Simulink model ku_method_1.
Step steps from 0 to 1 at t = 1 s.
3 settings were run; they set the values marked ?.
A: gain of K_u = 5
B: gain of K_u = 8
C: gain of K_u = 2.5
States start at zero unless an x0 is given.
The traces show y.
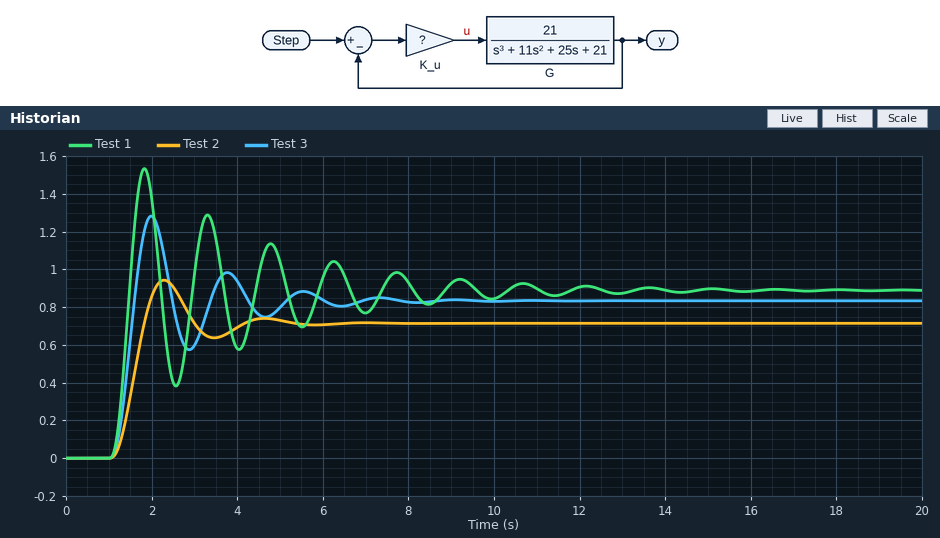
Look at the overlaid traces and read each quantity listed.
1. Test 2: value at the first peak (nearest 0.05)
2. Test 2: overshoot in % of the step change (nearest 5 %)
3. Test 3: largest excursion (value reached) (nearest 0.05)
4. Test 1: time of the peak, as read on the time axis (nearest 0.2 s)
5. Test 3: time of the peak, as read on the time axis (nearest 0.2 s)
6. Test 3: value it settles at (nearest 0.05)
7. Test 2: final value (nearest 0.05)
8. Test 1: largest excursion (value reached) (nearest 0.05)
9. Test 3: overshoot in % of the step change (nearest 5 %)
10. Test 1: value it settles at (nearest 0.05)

0.95
30 %
1.30
1.8 s
2.0 s
0.85
0.70
1.55
55 %
0.90
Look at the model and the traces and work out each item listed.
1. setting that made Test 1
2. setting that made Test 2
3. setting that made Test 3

B
C
A
